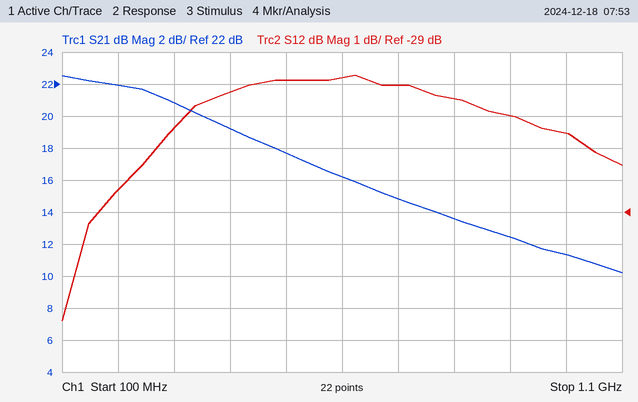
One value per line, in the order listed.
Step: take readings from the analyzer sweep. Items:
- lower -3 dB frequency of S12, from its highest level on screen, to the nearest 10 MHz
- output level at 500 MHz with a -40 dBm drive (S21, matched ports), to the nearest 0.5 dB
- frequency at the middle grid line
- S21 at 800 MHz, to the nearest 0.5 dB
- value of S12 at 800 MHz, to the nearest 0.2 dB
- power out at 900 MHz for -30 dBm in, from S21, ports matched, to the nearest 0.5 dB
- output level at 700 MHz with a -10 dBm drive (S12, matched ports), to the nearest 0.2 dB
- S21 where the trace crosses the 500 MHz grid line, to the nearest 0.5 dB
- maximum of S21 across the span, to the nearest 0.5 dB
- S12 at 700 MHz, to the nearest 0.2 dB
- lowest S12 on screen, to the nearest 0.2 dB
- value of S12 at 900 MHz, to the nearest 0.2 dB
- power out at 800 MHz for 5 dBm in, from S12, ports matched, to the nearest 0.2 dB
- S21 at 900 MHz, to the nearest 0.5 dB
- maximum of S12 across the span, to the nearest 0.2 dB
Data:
230 MHz
-22.5 dBm
600 MHz
13.5 dB
-25.4 dB
-17.5 dBm
-35.0 dBm
17.5 dB
22.5 dB
-25.0 dB
-32.4 dB
-26.0 dB
-20.4 dBm
12.5 dB
-24.8 dB
